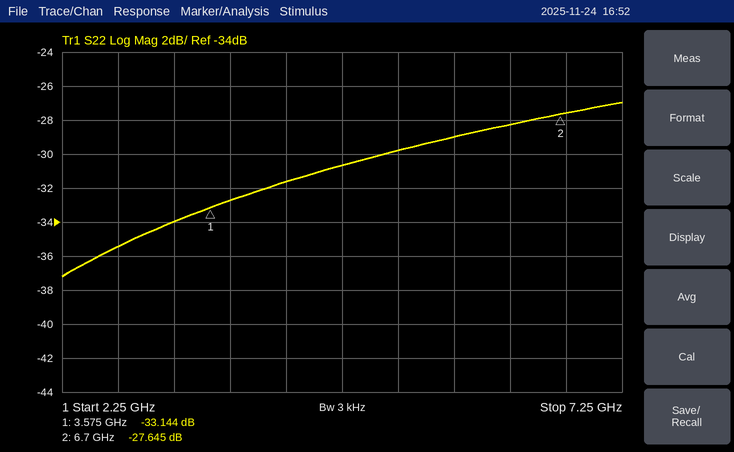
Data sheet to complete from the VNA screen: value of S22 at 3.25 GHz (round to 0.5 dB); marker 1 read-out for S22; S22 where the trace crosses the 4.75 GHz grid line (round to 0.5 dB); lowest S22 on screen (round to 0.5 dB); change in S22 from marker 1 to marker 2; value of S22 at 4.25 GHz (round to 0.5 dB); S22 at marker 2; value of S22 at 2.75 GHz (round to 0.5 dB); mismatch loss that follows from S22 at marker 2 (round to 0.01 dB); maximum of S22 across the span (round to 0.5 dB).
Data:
-34.0 dB
-33.144 dB
-30.5 dB
-37.0 dB
5.499 dB
-31.5 dB
-27.645 dB
-35.5 dB
0.01 dB
-27.0 dB
